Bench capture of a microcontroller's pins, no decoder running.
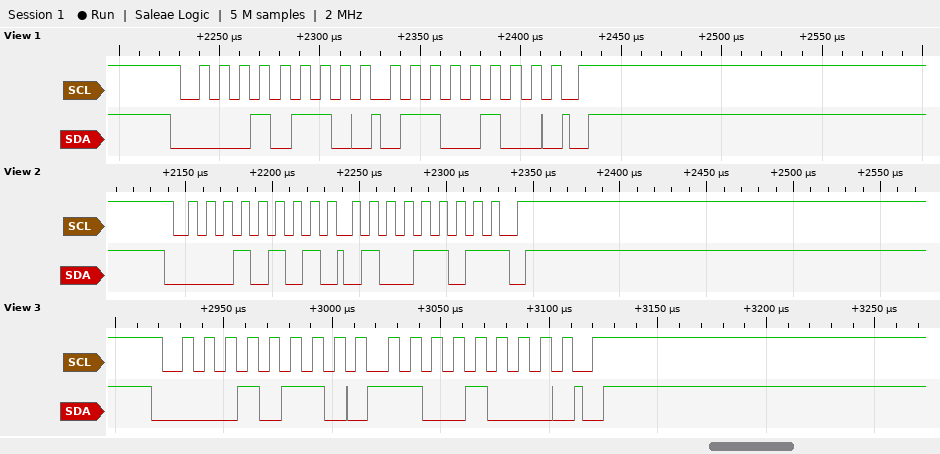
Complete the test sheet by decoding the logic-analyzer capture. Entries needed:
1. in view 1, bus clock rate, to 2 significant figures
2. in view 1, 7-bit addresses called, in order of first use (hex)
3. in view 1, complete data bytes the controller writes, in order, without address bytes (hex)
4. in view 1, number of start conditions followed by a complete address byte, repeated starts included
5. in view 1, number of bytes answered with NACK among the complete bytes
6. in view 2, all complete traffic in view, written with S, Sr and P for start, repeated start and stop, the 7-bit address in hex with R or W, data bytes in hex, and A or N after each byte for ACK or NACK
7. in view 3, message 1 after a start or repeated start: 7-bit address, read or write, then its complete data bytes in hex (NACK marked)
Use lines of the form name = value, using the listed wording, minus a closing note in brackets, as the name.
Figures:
in view 1, bus clock rate, to 2 significant figures = 100 kHz
in view 1, 7-bit addresses called, in order of first use = 0x0B
in view 1, complete data bytes the controller writes, in order, without address bytes = 64
in view 1, number of start conditions followed by a complete address byte, repeated starts included = 1
in view 1, number of bytes answered with NACK among the complete bytes = 0
in view 2, all complete traffic in view, written with S, Sr and P for start, repeated start and stop, the 7-bit address in hex with R or W, data bytes in hex, and A or N after each byte for ACK or NACK = S 0AR A 4D N P
in view 3, message 1 after a start or repeated start: 7-bit address, read or write, then its complete data bytes in hex = 0x0B write: C8
